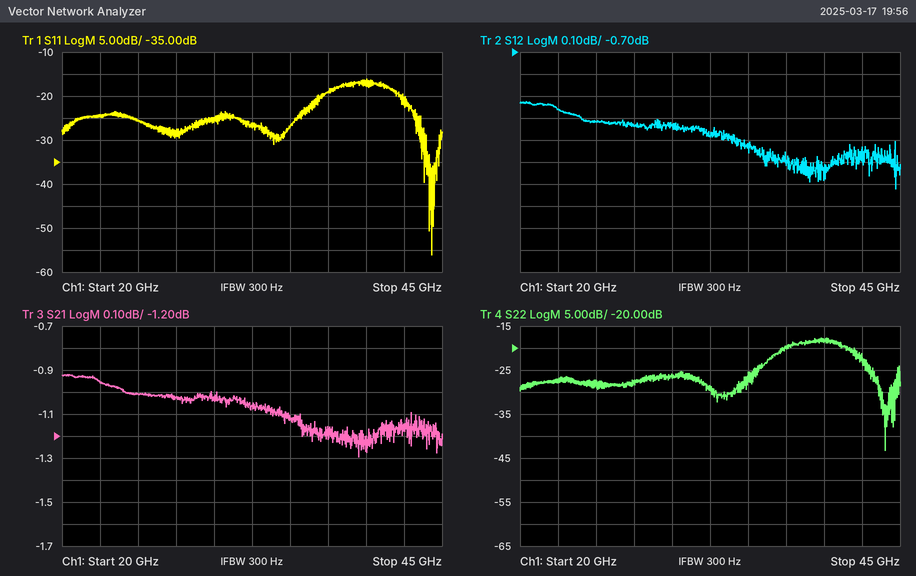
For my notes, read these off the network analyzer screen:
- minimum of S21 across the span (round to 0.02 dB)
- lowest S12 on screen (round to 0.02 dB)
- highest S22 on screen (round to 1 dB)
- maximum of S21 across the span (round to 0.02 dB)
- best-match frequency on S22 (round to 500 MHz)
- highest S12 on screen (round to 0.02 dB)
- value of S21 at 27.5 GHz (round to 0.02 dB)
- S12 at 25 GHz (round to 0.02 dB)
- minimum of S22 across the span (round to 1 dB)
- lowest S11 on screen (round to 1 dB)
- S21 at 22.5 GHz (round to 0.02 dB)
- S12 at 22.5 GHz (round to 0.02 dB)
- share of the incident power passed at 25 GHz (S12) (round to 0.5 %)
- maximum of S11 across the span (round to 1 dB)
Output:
-1.30 dB
-1.32 dB
-18 dB
-0.92 dB
44.0 GHz
-0.92 dB
-1.02 dB
-1.02 dB
-43 dB
-56 dB
-0.96 dB
-0.96 dB
79.0 %
-16 dB
